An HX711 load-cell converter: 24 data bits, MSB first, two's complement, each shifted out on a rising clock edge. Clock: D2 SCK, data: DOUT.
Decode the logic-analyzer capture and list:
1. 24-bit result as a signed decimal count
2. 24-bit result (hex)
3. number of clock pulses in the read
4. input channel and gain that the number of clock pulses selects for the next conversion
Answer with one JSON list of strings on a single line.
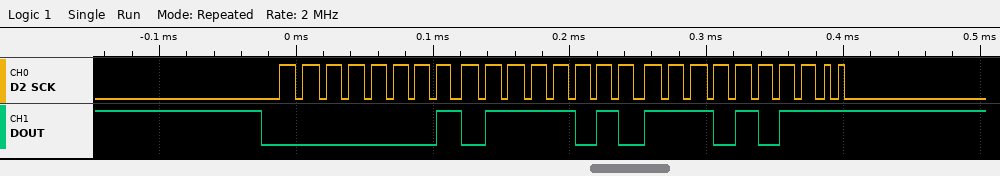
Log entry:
["97003", "0x017AEB", "26", "channel B, gain 32"]
